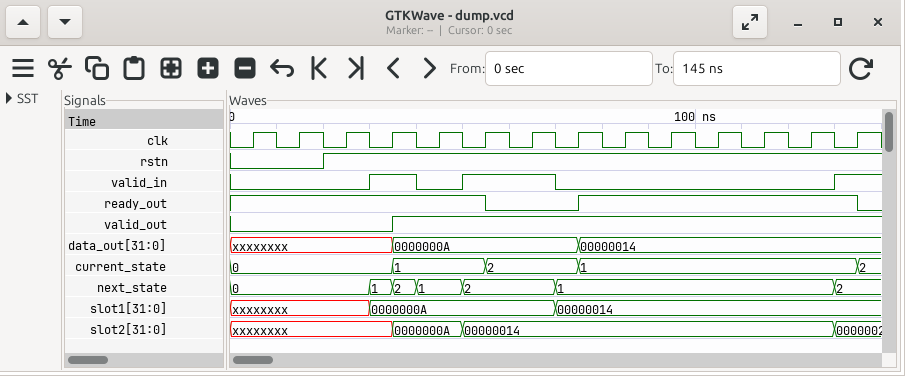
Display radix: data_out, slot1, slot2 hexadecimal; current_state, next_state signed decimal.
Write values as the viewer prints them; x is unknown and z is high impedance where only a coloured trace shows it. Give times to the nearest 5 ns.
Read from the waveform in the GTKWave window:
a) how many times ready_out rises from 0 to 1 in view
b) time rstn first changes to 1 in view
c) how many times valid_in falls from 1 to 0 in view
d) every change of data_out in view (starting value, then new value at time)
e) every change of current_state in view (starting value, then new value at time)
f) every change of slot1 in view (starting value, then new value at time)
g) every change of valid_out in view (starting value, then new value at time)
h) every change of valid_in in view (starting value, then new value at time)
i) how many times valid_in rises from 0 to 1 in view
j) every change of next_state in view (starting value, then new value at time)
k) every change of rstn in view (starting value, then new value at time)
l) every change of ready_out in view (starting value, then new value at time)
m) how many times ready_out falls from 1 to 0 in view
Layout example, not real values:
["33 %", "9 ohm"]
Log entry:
["1", "20 ns", "2", "xxxxxxxx, 0000000A at 35 ns, 00000014 at 75 ns", "0, 1 at 35 ns, 2 at 55 ns, 1 at 75 ns, 2 at 135 ns", "xxxxxxxx, 0000000A at 30 ns, 00000014 at 70 ns", "0, 1 at 35 ns", "0, 1 at 30 ns, 0 at 40 ns, 1 at 50 ns, 0 at 70 ns, 1 at 130 ns", "3", "0, 1 at 30 ns, 2 at 35 ns, 1 at 40 ns, 2 at 50 ns, 1 at 70 ns, 2 at 130 ns", "0, 1 at 20 ns", "1, 0 at 55 ns, 1 at 75 ns, 0 at 135 ns", "2"]
